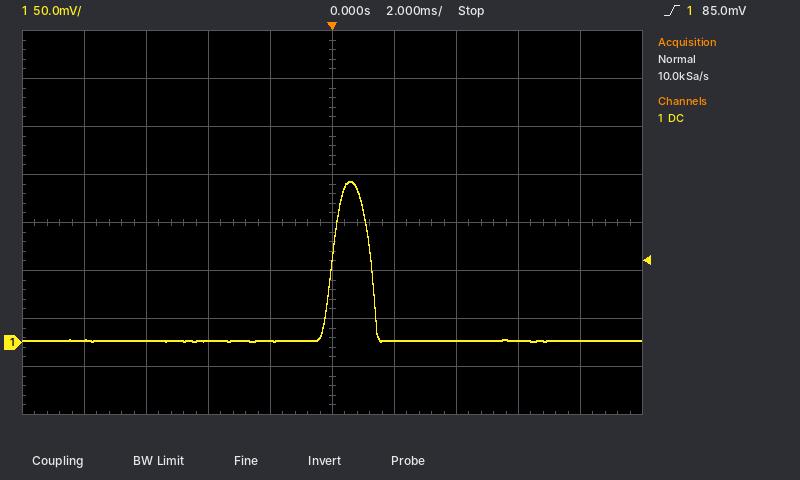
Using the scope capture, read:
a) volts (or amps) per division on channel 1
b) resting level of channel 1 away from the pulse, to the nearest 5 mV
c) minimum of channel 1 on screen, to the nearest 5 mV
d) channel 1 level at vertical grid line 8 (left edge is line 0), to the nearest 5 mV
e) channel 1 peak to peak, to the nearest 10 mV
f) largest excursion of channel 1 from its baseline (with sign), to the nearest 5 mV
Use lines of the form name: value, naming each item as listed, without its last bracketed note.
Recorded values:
volts (or amps) per division on channel 1: 50 mV
resting level of channel 1 away from the pulse, to the nearest 5 mV: 0 mV
minimum of channel 1 on screen, to the nearest 5 mV: 0 mV
channel 1 level at vertical grid line 8 (left edge is line 0), to the nearest 5 mV: 0 mV
channel 1 peak to peak, to the nearest 10 mV: 170 mV
largest excursion of channel 1 from its baseline (with sign), to the nearest 5 mV: +165 mV
